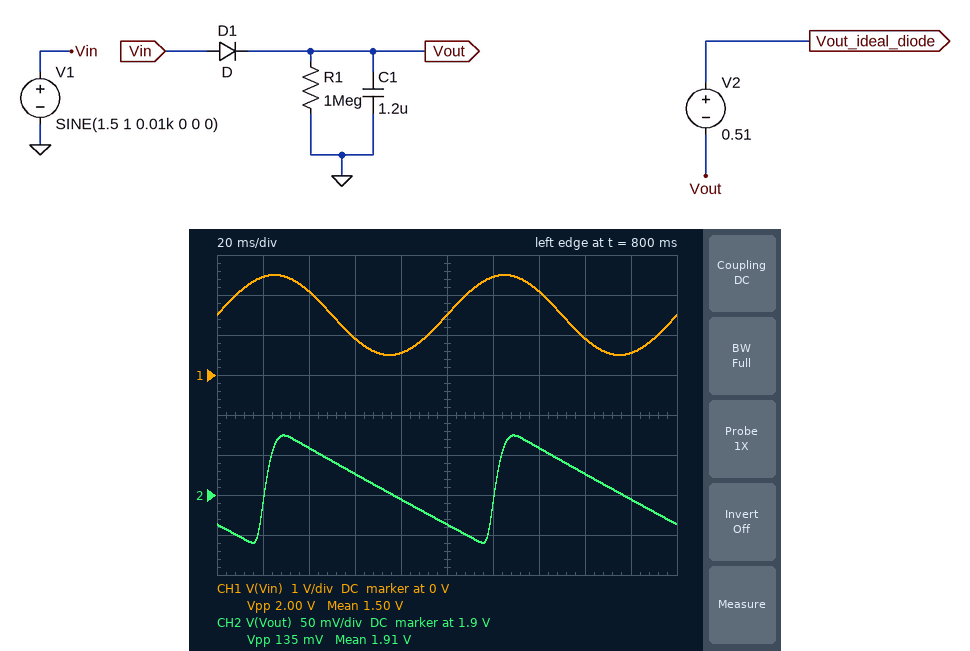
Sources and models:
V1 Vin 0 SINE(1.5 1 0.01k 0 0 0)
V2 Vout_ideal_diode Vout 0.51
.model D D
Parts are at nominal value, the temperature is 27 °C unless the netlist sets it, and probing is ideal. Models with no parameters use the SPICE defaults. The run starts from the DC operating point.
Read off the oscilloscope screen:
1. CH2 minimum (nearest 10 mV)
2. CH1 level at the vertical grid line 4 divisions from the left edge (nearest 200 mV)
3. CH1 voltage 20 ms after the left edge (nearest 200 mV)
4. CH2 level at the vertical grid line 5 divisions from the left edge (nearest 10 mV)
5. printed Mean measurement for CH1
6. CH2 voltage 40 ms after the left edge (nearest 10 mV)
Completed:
1.84 V
600 mV
2.4 V
1.86 V
1.50 V
1.96 V
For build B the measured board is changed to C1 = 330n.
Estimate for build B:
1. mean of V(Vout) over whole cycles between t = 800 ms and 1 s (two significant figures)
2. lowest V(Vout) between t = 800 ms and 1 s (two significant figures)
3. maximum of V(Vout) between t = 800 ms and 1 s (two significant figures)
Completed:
1.8 V
1.6 V
2.0 V
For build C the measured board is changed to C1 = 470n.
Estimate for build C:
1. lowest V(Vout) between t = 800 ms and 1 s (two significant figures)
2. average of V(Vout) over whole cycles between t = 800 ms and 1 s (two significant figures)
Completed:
1.7 V
1.8 V
